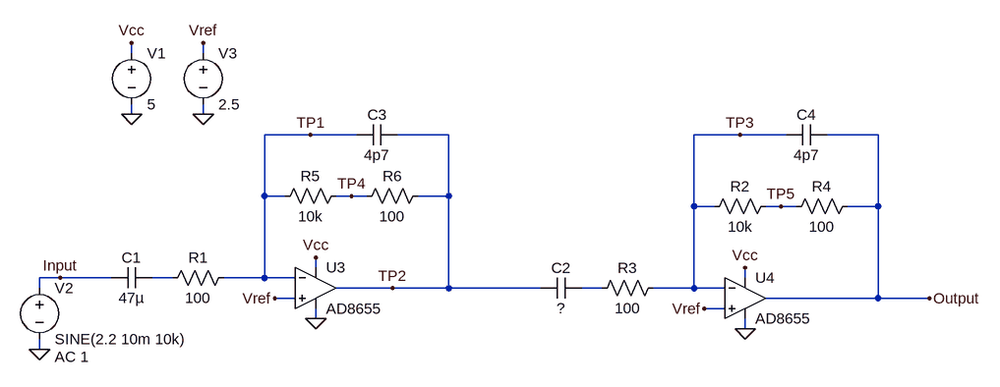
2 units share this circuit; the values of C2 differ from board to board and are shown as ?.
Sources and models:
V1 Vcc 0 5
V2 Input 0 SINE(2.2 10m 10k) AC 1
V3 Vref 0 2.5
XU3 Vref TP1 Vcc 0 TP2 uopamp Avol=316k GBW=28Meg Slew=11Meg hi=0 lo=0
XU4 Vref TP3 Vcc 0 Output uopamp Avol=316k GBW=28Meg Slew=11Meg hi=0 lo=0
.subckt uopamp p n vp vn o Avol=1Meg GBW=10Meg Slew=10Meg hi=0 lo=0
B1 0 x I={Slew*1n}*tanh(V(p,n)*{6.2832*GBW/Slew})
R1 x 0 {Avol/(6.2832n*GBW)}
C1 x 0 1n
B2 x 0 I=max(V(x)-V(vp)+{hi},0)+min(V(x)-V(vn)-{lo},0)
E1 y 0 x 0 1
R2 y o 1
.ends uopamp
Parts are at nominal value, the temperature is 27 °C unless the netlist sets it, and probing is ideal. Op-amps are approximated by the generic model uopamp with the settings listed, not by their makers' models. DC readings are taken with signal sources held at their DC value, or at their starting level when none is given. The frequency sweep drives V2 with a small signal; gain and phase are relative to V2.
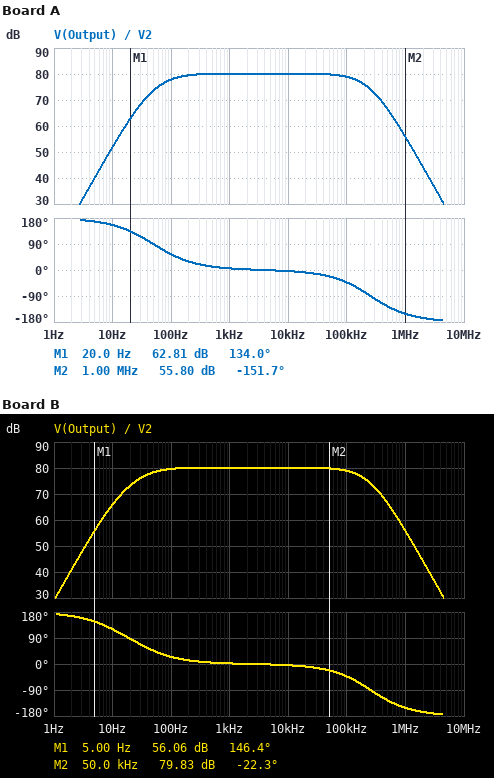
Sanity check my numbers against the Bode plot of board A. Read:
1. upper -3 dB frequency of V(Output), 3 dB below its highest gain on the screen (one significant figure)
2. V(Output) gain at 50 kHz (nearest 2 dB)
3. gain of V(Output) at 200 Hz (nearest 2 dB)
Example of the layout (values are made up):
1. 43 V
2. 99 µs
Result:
1. 200 kHz
2. 80 dB
3. 80 dB
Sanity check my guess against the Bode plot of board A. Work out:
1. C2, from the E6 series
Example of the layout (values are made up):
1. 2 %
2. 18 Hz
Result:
1. 22 µF
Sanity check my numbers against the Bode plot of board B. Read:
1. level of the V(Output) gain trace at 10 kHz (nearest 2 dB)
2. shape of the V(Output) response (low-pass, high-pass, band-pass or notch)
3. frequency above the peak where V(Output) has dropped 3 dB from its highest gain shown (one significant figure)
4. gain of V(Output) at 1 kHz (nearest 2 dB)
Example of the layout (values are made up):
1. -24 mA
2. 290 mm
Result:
1. 80 dB
2. band-pass
3. 200 kHz
4. 80 dB
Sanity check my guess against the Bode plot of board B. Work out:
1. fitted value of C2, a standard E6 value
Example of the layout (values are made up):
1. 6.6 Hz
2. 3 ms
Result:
1. 150 µF
